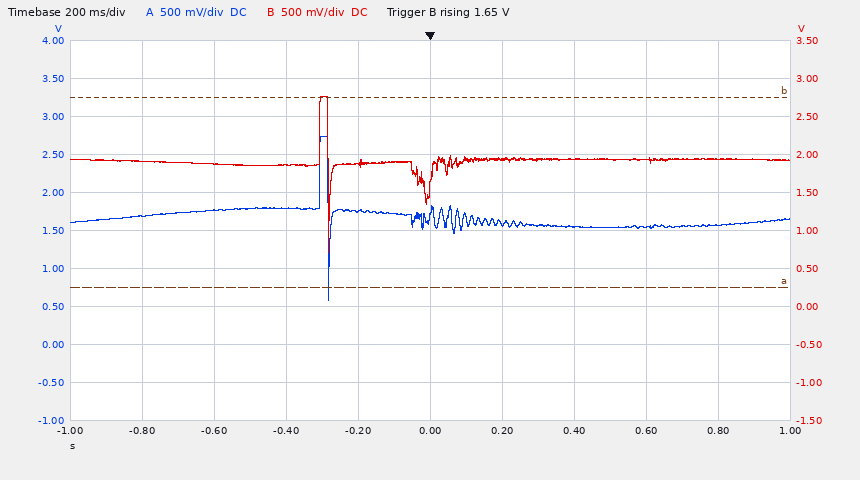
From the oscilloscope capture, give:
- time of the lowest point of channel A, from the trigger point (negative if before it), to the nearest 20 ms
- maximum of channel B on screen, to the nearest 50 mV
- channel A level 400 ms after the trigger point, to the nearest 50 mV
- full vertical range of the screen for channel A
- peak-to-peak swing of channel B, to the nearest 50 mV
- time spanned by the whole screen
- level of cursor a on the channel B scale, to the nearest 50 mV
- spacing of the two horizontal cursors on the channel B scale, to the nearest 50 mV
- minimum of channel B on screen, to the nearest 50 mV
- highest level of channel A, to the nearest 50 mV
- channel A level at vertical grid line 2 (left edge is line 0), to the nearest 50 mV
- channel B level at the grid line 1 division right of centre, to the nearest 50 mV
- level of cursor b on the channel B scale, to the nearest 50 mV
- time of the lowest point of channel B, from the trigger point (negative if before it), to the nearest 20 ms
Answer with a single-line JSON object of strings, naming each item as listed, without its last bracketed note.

{"time of the lowest point of channel A, from the trigger point (negative if before it), to the nearest 20 ms": "-280 ms", "maximum of channel B on screen, to the nearest 50 mV": "2.75 V", "channel A level 400 ms after the trigger point, to the nearest 50 mV": "1.55 V", "full vertical range of the screen for channel A": "5 V", "peak-to-peak swing of channel B, to the nearest 50 mV": "2.05 V", "time spanned by the whole screen": "2 s", "level of cursor a on the channel B scale, to the nearest 50 mV": "250 mV", "spacing of the two horizontal cursors on the channel B scale, to the nearest 50 mV": "2.50 V", "minimum of channel B on screen, to the nearest 50 mV": "700 mV", "highest level of channel A, to the nearest 50 mV": "2.75 V", "channel A level at vertical grid line 2 (left edge is line 0), to the nearest 50 mV": "1.75 V", "channel B level at the grid line 1 division right of centre, to the nearest 50 mV": "1.95 V", "level of cursor b on the channel B scale, to the nearest 50 mV": "2.75 V", "time of the lowest point of channel B, from the trigger point (negative if before it), to the nearest 20 ms": "-280 ms"}
